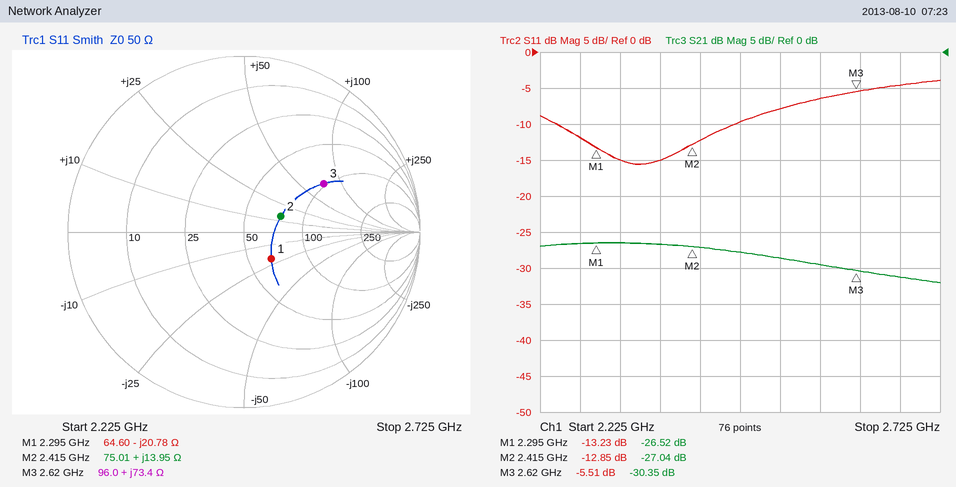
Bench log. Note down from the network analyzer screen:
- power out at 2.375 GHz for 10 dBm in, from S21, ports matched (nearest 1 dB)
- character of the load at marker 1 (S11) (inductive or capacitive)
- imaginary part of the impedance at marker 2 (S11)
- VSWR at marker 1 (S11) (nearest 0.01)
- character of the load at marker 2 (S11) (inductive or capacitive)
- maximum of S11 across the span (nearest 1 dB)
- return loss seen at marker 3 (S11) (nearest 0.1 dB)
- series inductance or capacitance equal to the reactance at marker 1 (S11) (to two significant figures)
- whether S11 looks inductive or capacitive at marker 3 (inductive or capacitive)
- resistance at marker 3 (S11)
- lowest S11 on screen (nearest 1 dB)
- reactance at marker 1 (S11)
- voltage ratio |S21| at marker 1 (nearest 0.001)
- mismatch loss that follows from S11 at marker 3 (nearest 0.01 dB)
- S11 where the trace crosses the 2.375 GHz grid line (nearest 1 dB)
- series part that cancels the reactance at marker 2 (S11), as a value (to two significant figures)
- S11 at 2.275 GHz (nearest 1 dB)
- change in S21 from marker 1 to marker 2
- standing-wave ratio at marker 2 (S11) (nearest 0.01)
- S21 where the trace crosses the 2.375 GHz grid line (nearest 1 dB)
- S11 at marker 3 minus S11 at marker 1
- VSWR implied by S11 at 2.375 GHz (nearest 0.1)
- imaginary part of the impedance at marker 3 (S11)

-17 dBm
capacitive
+13.95 Ω
1.56
inductive
-4 dB
5.5 dB
3.3 pF
inductive
96.0 Ω
-16 dB
-20.78 Ω
0.047
1.43 dB
-15 dB
4.7 pF
-12 dB
-0.52 dB
1.59
-27 dB
7.72 dB
1.4
+73.4 Ω
